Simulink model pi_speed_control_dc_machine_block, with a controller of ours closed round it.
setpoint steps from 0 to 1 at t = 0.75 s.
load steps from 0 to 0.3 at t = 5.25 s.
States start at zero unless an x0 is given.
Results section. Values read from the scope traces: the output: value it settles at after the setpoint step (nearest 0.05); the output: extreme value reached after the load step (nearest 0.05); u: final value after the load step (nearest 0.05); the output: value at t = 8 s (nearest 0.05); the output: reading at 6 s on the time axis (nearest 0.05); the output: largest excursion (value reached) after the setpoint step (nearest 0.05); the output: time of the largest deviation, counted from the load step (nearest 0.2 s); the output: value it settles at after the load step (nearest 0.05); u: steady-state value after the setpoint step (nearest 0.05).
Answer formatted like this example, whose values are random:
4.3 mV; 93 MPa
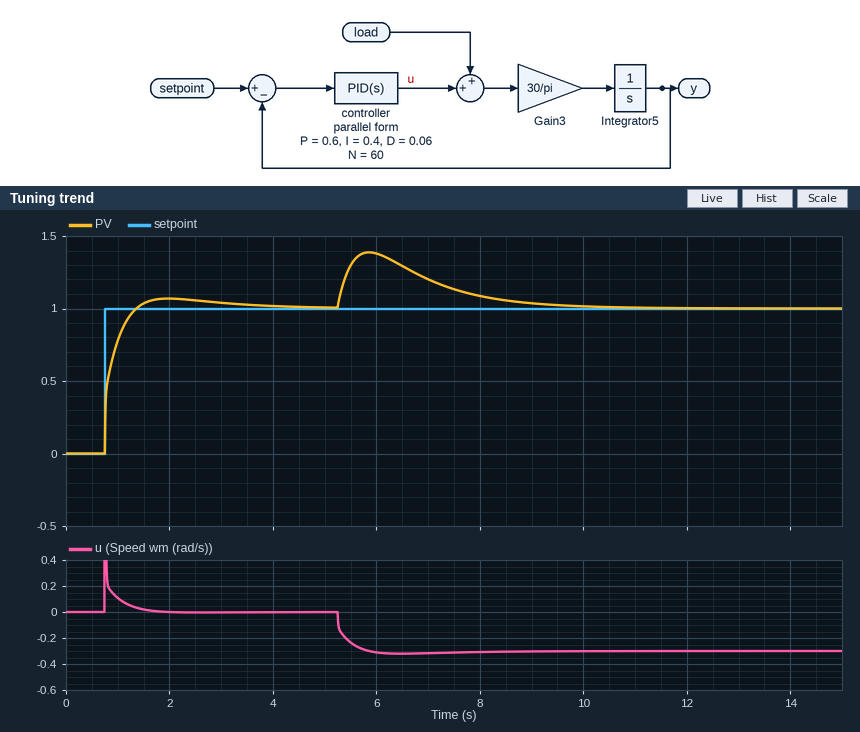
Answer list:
1.00; 1.40; -0.30; 1.10; 1.40; 1.05; 0.6 s; 1.00; 0.00
